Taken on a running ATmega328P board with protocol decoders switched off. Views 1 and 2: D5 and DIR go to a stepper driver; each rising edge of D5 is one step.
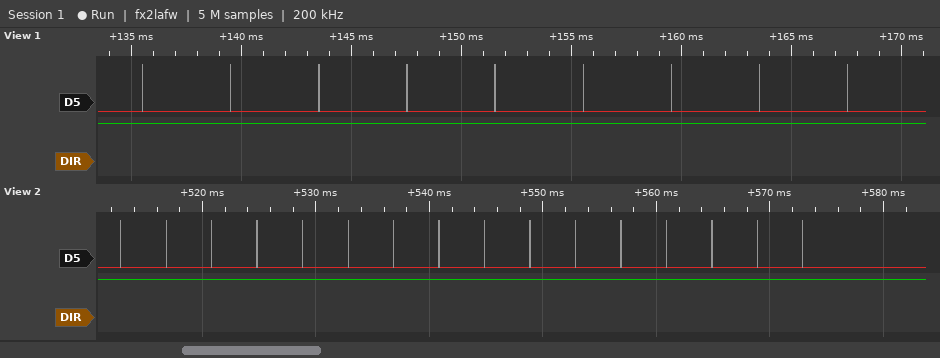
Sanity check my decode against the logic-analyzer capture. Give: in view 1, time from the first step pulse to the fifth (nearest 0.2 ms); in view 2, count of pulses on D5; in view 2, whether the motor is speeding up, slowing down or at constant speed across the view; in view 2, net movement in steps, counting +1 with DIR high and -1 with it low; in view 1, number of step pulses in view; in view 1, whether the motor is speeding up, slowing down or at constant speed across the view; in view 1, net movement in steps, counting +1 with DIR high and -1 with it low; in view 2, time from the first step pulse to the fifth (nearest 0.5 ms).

16.0 ms
16
constant speed
+16
9
constant speed
+9
16.0 ms
